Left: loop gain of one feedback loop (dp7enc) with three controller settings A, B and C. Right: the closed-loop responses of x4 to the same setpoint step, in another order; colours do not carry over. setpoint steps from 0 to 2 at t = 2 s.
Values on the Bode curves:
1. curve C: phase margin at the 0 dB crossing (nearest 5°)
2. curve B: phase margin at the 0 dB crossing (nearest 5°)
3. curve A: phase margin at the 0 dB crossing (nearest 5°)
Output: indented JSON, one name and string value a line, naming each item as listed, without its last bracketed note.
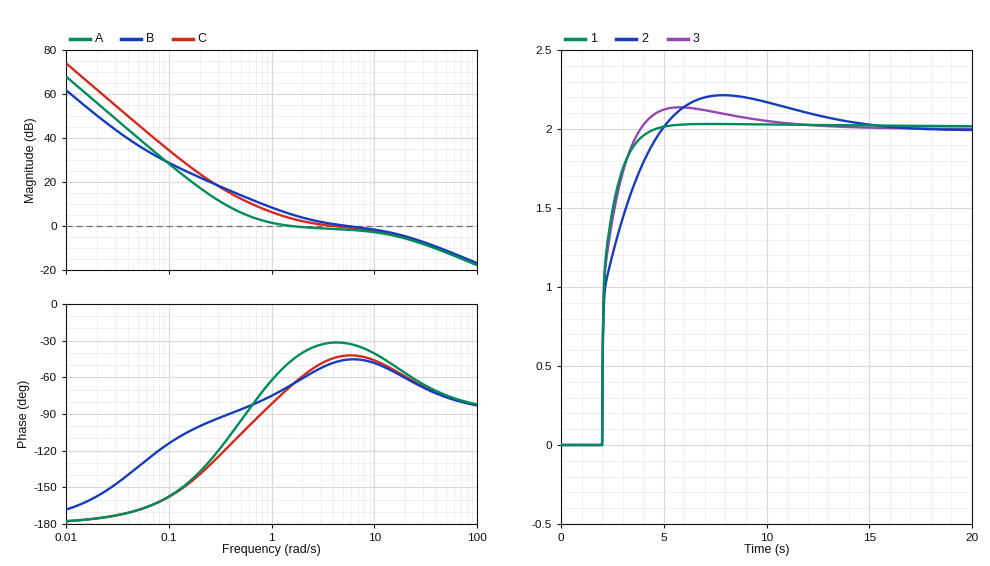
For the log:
{
  "curve C: phase margin at the 0 dB crossing": "135°",
  "curve B: phase margin at the 0 dB crossing": "135°",
  "curve A: phase margin at the 0 dB crossing": "135°"
}
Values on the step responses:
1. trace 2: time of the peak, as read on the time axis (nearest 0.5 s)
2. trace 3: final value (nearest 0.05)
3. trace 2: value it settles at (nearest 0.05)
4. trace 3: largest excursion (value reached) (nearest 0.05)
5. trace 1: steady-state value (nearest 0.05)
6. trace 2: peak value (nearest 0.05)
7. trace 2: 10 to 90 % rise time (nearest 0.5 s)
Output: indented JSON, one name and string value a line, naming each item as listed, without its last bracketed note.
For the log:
{
  "trace 2: time of the peak, as read on the time axis": "8.0 s",
  "trace 3: final value": "2.00",
  "trace 2: value it settles at": "2.00",
  "trace 3: largest excursion (value reached)": "2.15",
  "trace 1: steady-state value": "2.00",
  "trace 2: peak value": "2.20",
  "trace 2: 10 to 90 % rise time": "2.0 s"
}
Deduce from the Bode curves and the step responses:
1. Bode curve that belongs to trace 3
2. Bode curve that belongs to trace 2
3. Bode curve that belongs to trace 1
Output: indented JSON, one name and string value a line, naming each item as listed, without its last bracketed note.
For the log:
{
  "Bode curve that belongs to trace 3": "C",
  "Bode curve that belongs to trace 2": "A",
  "Bode curve that belongs to trace 1": "B"
}
